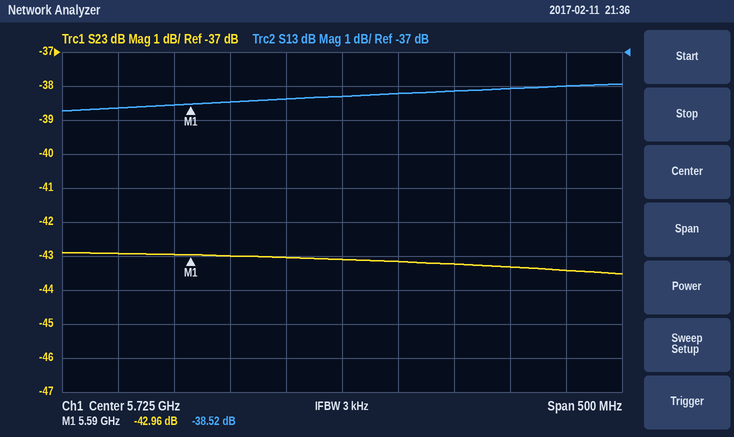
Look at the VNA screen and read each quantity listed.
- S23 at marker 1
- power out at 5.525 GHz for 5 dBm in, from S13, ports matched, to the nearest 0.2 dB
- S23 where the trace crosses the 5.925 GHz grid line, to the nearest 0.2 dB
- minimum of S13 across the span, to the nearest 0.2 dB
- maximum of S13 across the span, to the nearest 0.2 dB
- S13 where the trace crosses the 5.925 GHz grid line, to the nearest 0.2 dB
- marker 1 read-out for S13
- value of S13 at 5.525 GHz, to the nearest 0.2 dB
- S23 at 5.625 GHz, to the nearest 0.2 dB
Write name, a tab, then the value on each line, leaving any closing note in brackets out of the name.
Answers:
S23 at marker 1	-42.96 dB
power out at 5.525 GHz for 5 dBm in, from S13, ports matched, to the nearest 0.2 dB	-33.6 dBm
S23 where the trace crosses the 5.925 GHz grid line, to the nearest 0.2 dB	-43.4 dB
minimum of S13 across the span, to the nearest 0.2 dB	-38.8 dB
maximum of S13 across the span, to the nearest 0.2 dB	-38.0 dB
S13 where the trace crosses the 5.925 GHz grid line, to the nearest 0.2 dB	-38.0 dB
marker 1 read-out for S13	-38.52 dB
value of S13 at 5.525 GHz, to the nearest 0.2 dB	-38.6 dB
S23 at 5.625 GHz, to the nearest 0.2 dB	-43.0 dB
